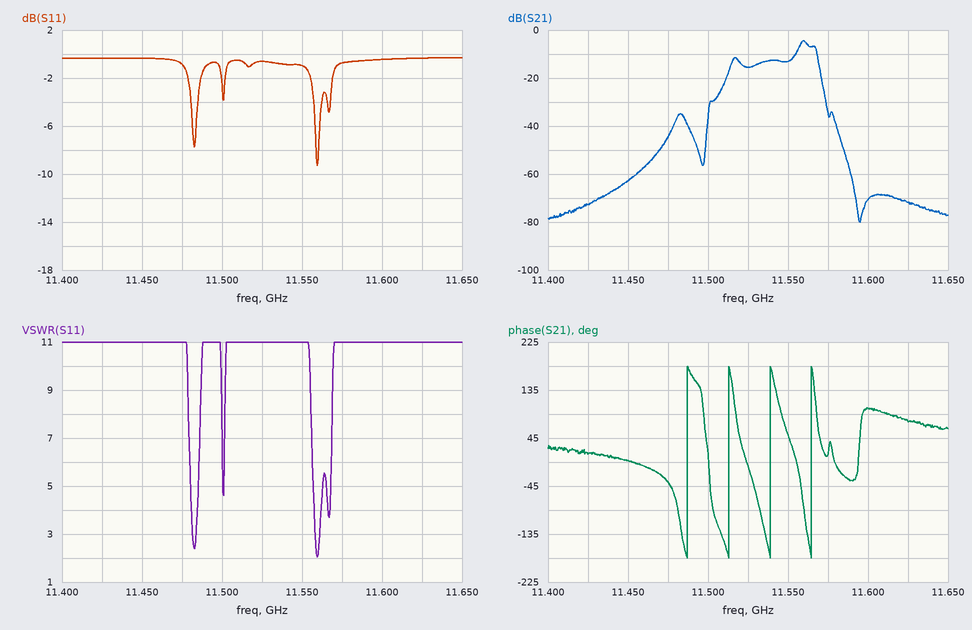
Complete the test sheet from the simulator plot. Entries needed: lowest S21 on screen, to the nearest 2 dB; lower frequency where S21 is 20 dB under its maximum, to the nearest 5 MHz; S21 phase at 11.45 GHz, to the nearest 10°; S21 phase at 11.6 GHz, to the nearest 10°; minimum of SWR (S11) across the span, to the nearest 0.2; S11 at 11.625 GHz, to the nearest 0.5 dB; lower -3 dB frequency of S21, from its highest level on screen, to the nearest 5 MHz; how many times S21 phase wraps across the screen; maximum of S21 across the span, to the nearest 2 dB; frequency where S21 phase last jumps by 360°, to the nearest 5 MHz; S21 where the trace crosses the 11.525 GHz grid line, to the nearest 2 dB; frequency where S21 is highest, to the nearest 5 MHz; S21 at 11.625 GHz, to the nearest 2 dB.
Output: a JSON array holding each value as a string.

["-80 dB", "11.510 GHz", "0°", "100°", "2.0", "-0.5 dB", "11.555 GHz", "4", "-4 dB", "11.565 GHz", "-16 dB", "11.560 GHz", "-72 dB"]
